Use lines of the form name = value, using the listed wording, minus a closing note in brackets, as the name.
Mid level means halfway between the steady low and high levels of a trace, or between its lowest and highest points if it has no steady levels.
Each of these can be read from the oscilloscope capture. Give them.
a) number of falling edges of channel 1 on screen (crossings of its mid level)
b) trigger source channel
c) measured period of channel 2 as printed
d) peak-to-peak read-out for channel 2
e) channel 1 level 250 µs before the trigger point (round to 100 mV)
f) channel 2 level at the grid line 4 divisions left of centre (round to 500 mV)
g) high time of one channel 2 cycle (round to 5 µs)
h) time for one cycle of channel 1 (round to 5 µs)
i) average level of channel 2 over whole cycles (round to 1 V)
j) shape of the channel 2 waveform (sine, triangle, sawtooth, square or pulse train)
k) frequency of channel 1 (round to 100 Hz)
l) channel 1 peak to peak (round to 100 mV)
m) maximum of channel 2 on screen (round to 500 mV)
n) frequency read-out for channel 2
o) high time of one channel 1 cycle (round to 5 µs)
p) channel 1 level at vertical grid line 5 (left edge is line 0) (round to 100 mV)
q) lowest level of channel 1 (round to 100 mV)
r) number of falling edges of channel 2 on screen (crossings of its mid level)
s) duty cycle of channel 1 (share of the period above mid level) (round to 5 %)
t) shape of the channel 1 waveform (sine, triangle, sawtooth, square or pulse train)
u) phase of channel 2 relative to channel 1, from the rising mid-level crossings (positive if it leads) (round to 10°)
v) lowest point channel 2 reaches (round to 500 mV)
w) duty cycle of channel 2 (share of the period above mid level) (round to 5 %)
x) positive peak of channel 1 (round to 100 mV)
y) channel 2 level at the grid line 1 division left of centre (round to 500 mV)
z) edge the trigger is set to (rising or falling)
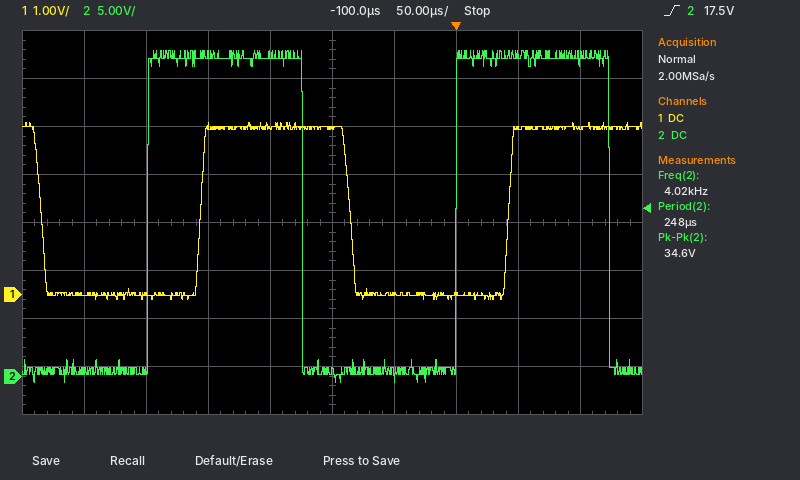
number of falling edges of channel 1 on screen = 2
trigger source channel = channel 2
measured period of channel 2 as printed = 248 µs
peak-to-peak read-out for channel 2 = 34.6 V
channel 1 level 250 µs before the trigger point = 0.0 V
channel 2 level at the grid line 4 divisions left of centre = 500 mV
high time of one channel 2 cycle = 125 µs
time for one cycle of channel 1 = 250 µs
average level of channel 2 over whole cycles = 17 V
shape of the channel 2 waveform = square
frequency of channel 1 = 4.0 kHz
channel 1 peak to peak = 3.7 V
maximum of channel 2 on screen = 34.0 V
frequency read-out for channel 2 = 4.02 kHz
high time of one channel 1 cycle = 120 µs
channel 1 level at vertical grid line 5 (left edge is line 0) = 3.5 V
lowest level of channel 1 = -100 mV
number of falling edges of channel 2 on screen = 2
duty cycle of channel 1 (share of the period above mid level) = 50 %
shape of the channel 1 waveform = square
phase of channel 2 relative to channel 1, from the rising mid-level crossings (positive if it leads) = +60°
lowest point channel 2 reaches = -500 mV
duty cycle of channel 2 (share of the period above mid level) = 50 %
positive peak of channel 1 = 3.6 V
channel 2 level at the grid line 1 division left of centre = 33.5 V
edge the trigger is set to = rising
